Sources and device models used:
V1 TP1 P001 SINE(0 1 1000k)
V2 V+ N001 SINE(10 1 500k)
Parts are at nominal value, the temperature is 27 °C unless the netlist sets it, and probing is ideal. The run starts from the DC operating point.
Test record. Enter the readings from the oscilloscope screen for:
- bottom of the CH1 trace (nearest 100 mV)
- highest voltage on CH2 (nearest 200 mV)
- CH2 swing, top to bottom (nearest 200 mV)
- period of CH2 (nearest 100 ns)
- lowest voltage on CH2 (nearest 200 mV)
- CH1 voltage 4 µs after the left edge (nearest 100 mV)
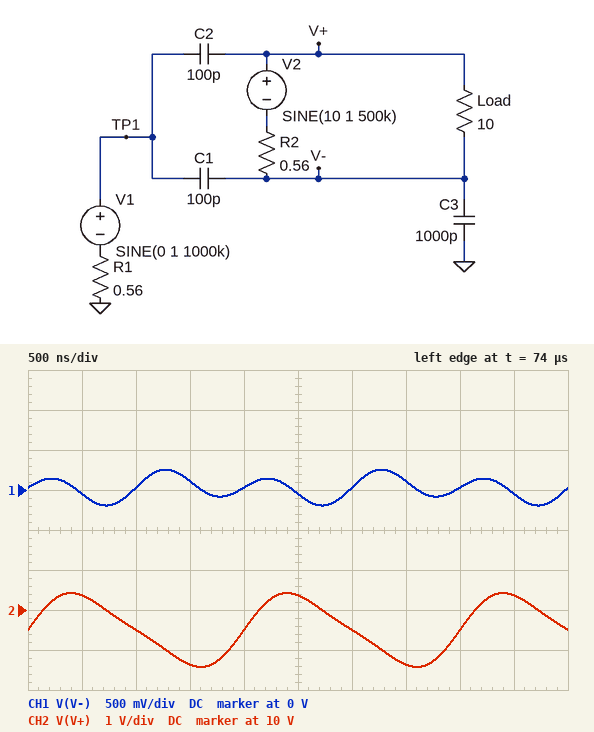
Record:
-200 mV
10.4 V
1.8 V
2.0 µs
8.6 V
0 V
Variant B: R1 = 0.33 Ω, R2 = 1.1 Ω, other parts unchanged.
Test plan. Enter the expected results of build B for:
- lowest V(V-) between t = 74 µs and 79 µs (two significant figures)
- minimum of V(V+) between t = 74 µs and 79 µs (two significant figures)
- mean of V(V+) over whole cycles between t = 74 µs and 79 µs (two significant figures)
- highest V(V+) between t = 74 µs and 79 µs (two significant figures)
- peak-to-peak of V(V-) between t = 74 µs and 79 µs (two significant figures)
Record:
-970 mV
7.4 V
8.3 V
9.1 V
440 mV
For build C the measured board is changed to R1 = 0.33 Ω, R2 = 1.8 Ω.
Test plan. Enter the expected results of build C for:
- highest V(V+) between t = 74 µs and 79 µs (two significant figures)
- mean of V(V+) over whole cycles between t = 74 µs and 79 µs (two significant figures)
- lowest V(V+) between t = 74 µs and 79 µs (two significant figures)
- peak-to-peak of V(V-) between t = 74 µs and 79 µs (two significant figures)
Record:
8.6 V
7.8 V
6.9 V
440 mV
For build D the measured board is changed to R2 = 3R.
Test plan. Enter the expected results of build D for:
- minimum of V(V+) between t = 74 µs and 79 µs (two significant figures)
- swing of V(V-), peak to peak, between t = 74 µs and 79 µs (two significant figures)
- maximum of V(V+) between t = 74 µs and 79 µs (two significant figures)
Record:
6.3 V
430 mV
7.8 V
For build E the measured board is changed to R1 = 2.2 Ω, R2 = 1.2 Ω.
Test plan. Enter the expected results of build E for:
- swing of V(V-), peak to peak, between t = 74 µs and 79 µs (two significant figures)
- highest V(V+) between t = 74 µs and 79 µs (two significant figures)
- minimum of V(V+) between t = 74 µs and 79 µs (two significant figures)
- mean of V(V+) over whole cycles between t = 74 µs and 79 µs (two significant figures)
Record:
440 mV
9.1 V
7.3 V
8.2 V
